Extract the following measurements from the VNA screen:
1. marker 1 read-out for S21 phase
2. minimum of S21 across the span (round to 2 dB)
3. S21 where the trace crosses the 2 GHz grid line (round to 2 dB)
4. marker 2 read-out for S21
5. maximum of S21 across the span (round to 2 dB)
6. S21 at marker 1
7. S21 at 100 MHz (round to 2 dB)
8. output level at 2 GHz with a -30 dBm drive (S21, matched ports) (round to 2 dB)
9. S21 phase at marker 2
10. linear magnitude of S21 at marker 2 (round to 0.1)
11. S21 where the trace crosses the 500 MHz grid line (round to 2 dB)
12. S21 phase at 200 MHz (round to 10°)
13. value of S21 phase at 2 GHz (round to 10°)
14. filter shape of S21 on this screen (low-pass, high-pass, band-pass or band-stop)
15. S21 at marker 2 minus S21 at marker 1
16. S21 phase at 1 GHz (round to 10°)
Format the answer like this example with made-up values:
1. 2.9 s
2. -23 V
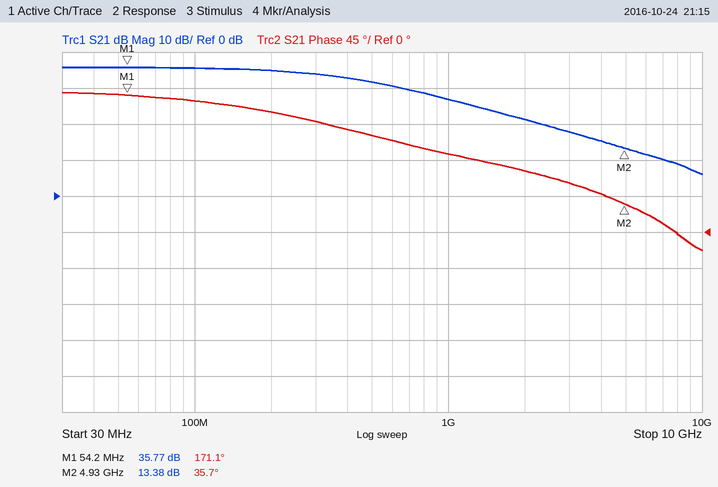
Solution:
1. 171.1°
2. 6 dB
3. 22 dB
4. 13.38 dB
5. 36 dB
6. 35.77 dB
7. 36 dB
8. -8 dBm
9. 35.7°
10. 4.7
11. 32 dB
12. 150°
13. 80°
14. low-pass
15. -22.39 dB
16. 100°
